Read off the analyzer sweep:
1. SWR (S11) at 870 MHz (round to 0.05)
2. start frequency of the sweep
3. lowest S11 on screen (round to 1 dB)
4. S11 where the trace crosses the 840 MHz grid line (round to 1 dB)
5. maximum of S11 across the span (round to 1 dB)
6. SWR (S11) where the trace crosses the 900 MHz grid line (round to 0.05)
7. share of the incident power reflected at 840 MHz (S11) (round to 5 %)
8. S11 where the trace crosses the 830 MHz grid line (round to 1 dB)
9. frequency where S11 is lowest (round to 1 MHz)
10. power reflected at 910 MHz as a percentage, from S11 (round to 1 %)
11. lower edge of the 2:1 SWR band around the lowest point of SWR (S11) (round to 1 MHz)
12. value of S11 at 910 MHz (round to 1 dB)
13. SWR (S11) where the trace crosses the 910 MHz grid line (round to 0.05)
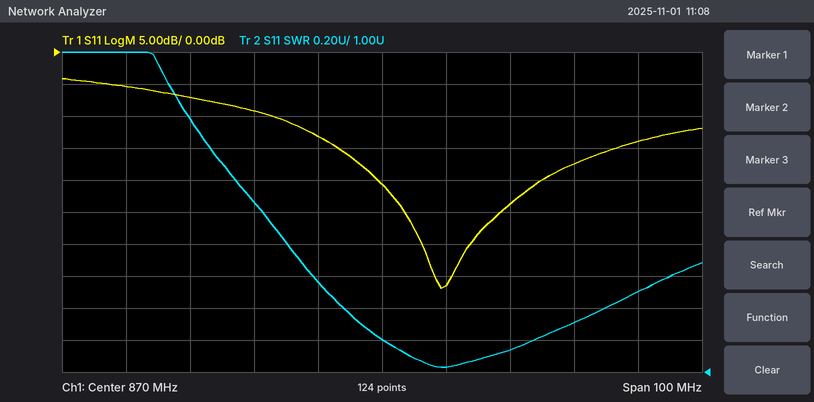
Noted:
1.20
820 MHz
-37 dB
-7 dB
-4 dB
1.30
20 %
-5 dB
879 MHz
4 %
851 MHz
-14 dB
1.50
